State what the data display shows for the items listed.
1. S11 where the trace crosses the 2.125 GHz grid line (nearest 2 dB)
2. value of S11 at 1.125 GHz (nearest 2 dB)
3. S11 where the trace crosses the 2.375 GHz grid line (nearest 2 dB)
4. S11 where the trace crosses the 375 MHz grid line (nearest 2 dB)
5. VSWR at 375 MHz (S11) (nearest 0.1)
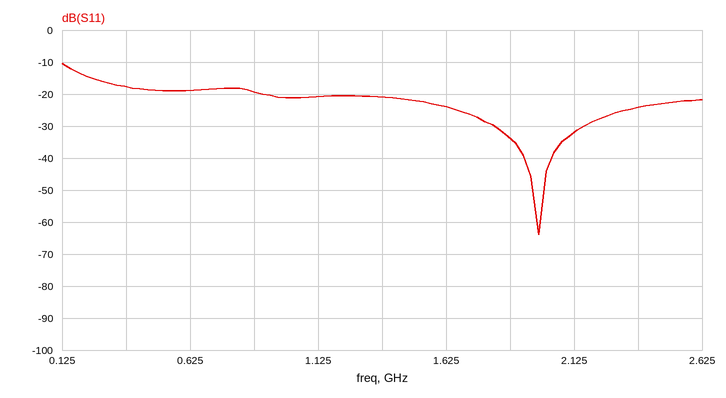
-32 dB
-20 dB
-24 dB
-18 dB
1.3
